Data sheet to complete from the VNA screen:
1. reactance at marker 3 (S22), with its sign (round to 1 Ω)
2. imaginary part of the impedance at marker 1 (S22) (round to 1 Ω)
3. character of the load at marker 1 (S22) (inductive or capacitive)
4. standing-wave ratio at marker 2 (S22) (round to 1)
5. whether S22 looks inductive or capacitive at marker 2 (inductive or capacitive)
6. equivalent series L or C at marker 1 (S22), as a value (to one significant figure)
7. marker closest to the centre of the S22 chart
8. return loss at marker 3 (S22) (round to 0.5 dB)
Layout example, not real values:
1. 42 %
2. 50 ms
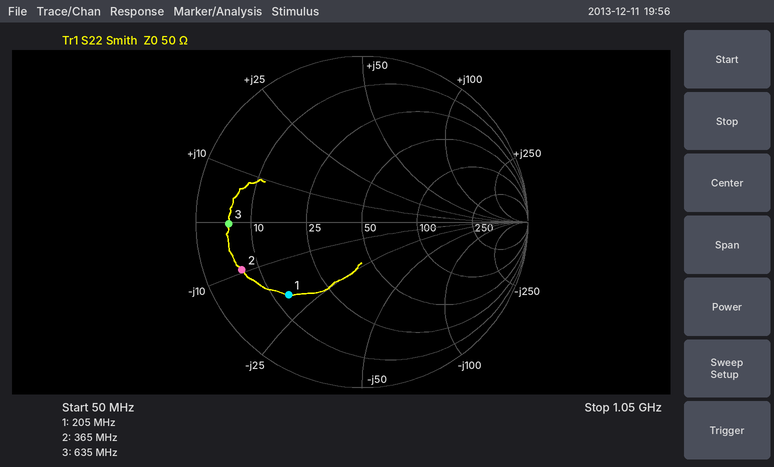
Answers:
1. 0 Ω
2. -19 Ω
3. capacitive
4. 8
5. capacitive
6. 40 pF
7. marker 1
8. 2.0 dB
